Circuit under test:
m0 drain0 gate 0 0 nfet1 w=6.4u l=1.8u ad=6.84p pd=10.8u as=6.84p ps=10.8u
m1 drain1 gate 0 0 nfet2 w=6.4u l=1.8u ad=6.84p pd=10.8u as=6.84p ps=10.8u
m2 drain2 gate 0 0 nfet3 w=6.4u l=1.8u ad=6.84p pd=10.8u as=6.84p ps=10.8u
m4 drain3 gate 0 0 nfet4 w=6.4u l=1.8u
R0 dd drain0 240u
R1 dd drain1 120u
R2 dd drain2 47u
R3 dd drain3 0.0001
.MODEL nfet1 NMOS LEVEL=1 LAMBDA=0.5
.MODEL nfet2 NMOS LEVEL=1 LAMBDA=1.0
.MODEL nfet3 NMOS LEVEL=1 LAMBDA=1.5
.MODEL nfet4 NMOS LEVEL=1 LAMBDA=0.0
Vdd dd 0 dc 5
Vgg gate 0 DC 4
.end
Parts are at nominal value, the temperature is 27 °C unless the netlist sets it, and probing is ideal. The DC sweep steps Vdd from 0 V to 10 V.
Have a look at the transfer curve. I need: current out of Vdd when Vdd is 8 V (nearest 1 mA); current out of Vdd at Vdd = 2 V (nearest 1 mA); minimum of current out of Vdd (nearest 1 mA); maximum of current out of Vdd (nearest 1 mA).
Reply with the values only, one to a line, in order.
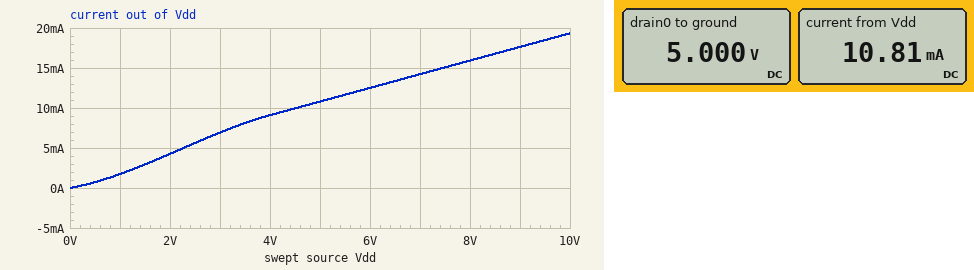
16 mA
4 mA
0 A
19 mA
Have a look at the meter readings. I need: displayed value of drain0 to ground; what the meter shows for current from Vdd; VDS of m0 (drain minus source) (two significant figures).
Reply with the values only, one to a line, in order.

5.000 V
10.81 mA
5.0 V
